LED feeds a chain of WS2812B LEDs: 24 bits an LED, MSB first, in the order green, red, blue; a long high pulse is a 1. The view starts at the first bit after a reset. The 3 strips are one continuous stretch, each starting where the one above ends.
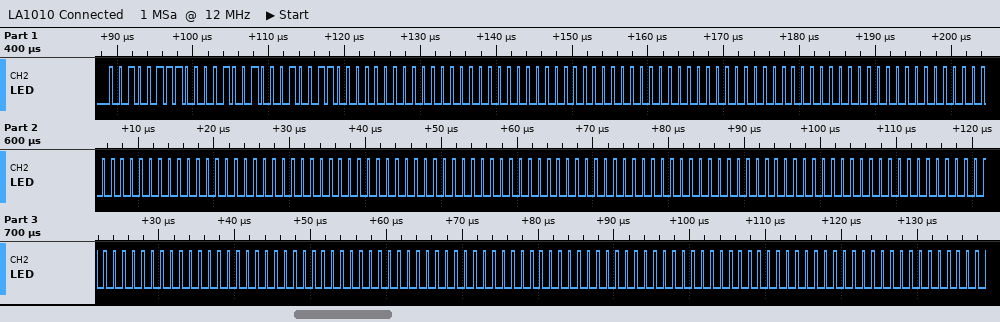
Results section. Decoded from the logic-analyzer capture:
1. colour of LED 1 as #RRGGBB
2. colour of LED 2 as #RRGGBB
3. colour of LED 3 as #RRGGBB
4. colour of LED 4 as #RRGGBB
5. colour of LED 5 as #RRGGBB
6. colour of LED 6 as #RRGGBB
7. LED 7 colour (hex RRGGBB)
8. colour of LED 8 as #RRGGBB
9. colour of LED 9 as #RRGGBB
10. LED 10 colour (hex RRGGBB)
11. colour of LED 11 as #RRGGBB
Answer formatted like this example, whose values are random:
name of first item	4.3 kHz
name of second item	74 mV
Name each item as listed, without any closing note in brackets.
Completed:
colour of LED 1 as #RRGGBB	#092713
colour of LED 2 as #RRGGBB	#000000
colour of LED 3 as #RRGGBB	#000000
colour of LED 4 as #RRGGBB	#000000
colour of LED 5 as #RRGGBB	#000000
colour of LED 6 as #RRGGBB	#000000
LED 7 colour	#000000
colour of LED 8 as #RRGGBB	#000000
colour of LED 9 as #RRGGBB	#000000
LED 10 colour	#000000
colour of LED 11 as #RRGGBB	#000000
